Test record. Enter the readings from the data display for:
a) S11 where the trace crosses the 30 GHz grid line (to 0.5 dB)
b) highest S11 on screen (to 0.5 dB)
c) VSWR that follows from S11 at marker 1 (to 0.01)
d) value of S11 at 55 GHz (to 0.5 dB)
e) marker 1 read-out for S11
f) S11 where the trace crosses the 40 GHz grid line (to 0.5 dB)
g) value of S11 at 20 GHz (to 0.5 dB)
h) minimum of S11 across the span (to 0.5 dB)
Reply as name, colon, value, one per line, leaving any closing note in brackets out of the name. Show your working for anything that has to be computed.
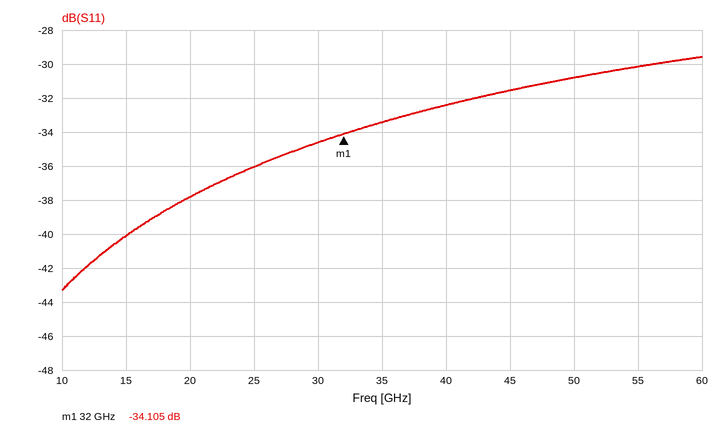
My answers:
S11 where the trace crosses the 30 GHz grid line: -34.5 dB
highest S11 on screen: -29.5 dB
VSWR that follows from S11 at marker 1: (1 + 0.0197)/(1 − 0.0197) ≈ 1.04
value of S11 at 55 GHz: -30.0 dB
marker 1 read-out for S11: -34.105 dB
S11 where the trace crosses the 40 GHz grid line: -32.5 dB
value of S11 at 20 GHz: -38.0 dB
minimum of S11 across the span: -43.5 dB
